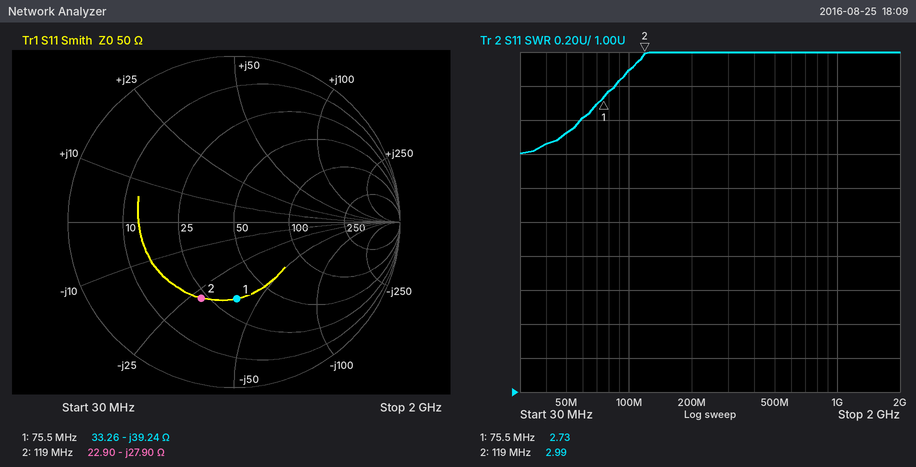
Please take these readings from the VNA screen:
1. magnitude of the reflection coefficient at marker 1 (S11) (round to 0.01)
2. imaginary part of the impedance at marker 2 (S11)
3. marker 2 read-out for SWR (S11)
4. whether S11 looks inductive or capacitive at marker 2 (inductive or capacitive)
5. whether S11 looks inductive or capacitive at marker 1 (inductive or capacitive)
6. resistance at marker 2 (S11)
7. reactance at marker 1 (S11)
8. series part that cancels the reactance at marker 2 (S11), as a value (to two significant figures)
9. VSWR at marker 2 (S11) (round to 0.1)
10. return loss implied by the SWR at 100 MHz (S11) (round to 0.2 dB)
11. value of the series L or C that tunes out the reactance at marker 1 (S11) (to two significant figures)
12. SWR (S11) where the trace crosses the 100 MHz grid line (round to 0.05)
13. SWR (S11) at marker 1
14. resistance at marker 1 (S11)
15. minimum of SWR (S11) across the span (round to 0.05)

0.46
-27.90 Ω
2.99
capacitive
capacitive
22.90 Ω
-39.24 Ω
37 nH
3.0
6.2 dB
83 nH
2.90
2.73
33.26 Ω
2.40
